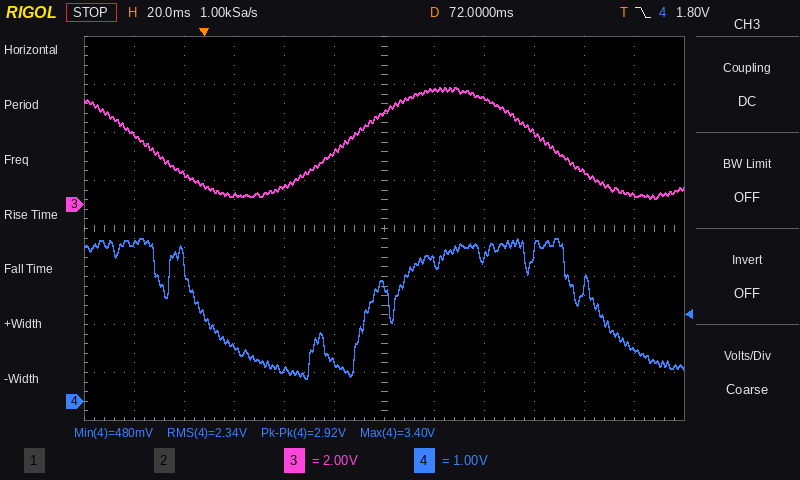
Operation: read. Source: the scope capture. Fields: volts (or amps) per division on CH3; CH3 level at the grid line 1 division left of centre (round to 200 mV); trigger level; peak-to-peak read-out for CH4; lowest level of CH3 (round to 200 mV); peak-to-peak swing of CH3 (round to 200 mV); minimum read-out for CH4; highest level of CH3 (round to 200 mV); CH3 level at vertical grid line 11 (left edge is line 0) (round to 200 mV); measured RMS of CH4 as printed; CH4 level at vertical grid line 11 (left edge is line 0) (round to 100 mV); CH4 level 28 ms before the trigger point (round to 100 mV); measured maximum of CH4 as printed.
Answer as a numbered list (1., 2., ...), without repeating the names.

1. 2 V
2. 2.2 V
3. 1.80 V
4. 2.92 V
5. 200 mV
6. 4.6 V
7. 480 mV
8. 4.8 V
9. 400 mV
10. 2.34 V
11. 1.1 V
12. 3.3 V
13. 3.40 V
